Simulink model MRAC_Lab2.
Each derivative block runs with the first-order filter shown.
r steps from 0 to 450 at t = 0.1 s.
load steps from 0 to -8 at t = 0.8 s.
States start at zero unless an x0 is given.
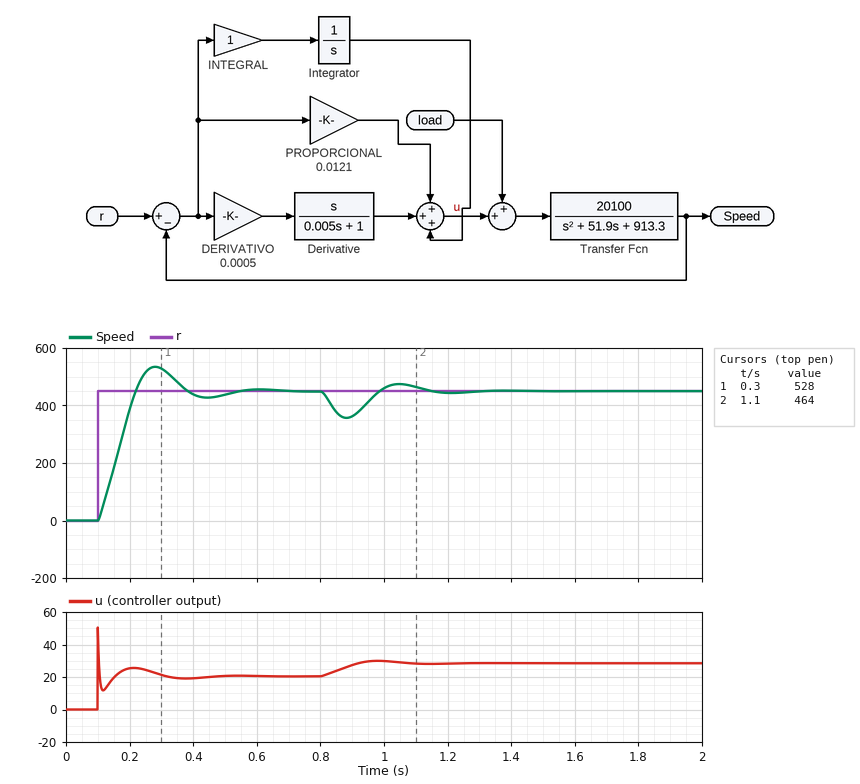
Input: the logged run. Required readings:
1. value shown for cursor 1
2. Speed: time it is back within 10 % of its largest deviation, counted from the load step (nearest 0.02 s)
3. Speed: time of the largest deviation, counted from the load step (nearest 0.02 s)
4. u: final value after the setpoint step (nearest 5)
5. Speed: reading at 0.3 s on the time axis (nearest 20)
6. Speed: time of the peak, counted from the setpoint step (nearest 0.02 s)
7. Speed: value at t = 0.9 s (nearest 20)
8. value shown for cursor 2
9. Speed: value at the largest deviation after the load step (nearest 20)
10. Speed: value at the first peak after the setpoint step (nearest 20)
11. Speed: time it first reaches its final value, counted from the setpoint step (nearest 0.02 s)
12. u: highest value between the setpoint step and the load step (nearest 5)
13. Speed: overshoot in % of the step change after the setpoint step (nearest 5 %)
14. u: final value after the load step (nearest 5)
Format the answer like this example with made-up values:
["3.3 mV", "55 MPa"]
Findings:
["528", "0.32 s", "0.08 s", "20", "520", "0.18 s", "360", "464", "360", "540", "0.12 s", "50", "20 %", "30"]
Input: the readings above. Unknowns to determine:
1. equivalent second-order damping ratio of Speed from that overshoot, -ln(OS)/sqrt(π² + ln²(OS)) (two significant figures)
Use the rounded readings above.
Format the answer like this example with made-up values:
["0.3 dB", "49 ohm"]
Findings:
["0.46"]
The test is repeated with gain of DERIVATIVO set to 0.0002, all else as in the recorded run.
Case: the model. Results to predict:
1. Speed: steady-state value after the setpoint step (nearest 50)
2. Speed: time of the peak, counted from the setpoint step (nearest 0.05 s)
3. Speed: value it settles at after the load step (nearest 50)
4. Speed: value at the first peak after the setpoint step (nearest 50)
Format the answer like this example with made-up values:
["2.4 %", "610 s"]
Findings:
["450", "0.15 s", "450", "550"]
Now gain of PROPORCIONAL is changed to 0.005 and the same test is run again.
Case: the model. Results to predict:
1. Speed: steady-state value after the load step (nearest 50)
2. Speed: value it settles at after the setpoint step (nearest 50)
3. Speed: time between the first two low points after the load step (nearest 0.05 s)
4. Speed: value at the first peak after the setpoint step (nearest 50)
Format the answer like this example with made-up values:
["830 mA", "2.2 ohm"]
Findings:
["450", "450", "0.35 s", "550"]
